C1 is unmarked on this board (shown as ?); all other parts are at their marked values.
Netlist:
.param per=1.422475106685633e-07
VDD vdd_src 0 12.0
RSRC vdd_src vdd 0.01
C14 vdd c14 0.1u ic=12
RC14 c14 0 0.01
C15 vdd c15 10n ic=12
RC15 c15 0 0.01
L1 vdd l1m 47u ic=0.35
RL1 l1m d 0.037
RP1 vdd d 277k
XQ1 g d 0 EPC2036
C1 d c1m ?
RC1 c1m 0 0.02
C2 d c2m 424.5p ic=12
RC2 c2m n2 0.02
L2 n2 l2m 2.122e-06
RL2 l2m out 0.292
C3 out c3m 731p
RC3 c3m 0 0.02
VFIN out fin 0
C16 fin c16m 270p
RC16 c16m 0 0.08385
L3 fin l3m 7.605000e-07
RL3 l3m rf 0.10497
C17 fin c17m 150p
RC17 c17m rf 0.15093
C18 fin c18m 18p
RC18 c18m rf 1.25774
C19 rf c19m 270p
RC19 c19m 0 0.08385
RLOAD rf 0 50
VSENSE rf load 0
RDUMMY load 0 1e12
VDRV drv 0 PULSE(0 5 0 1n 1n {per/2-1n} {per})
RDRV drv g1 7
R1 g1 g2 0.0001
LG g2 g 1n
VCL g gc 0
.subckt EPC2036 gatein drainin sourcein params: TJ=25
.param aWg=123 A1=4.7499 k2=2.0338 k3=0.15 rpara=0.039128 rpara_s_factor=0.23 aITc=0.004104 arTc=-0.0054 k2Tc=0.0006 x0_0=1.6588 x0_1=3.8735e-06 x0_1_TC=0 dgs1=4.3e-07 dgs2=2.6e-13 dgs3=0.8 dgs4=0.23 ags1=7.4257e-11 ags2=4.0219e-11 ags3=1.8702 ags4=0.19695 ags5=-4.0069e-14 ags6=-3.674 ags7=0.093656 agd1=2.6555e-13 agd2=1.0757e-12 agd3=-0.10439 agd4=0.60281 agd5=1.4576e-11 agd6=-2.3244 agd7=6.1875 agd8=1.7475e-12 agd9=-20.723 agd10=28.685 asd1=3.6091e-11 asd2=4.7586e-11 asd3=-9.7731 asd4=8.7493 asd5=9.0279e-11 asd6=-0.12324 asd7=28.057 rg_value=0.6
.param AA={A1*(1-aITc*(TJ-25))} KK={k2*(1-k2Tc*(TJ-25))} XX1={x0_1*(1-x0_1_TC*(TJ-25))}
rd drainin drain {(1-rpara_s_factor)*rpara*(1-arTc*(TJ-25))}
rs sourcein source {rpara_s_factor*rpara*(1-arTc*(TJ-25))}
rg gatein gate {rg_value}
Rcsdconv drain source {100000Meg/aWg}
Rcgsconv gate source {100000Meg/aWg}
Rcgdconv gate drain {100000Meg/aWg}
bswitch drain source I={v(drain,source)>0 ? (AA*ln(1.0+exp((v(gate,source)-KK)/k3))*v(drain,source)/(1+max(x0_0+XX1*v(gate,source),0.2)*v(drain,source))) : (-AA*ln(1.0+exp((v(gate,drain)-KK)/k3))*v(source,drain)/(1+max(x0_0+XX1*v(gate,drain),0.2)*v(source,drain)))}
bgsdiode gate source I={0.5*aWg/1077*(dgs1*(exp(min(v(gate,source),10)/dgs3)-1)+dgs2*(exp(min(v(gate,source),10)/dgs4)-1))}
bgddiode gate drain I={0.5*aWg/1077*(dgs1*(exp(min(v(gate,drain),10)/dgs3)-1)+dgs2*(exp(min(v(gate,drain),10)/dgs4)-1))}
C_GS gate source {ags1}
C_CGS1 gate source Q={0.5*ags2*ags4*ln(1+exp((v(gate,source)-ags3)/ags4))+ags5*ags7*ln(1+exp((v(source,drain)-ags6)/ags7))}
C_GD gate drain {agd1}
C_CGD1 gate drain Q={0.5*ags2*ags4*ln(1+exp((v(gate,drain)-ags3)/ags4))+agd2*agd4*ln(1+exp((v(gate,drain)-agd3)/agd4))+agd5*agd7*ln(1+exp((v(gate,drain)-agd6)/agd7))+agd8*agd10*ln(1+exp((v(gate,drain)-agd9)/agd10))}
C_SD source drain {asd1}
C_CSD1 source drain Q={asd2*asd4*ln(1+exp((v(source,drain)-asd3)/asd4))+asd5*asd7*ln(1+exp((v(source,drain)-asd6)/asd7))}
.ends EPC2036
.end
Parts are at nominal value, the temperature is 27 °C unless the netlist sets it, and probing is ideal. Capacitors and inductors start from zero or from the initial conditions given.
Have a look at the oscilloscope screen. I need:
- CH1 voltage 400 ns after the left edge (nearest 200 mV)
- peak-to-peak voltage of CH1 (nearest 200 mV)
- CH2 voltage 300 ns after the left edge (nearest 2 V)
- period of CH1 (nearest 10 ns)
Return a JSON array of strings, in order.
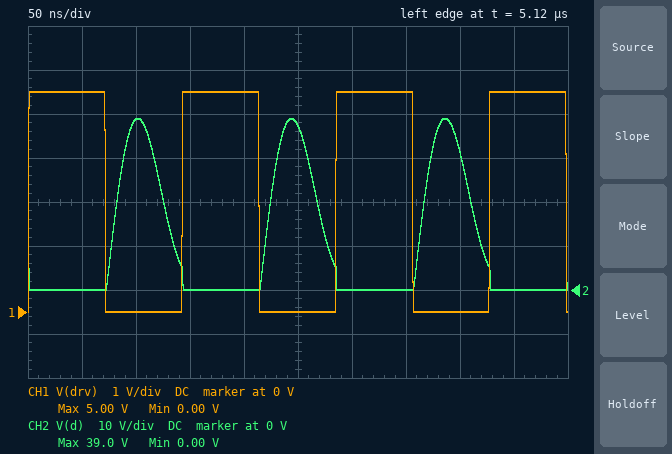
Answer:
["0 V", "5.0 V", "0 V", "140 ns"]
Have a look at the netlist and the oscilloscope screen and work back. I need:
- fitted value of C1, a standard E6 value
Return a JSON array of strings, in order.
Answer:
["330 pF"]
